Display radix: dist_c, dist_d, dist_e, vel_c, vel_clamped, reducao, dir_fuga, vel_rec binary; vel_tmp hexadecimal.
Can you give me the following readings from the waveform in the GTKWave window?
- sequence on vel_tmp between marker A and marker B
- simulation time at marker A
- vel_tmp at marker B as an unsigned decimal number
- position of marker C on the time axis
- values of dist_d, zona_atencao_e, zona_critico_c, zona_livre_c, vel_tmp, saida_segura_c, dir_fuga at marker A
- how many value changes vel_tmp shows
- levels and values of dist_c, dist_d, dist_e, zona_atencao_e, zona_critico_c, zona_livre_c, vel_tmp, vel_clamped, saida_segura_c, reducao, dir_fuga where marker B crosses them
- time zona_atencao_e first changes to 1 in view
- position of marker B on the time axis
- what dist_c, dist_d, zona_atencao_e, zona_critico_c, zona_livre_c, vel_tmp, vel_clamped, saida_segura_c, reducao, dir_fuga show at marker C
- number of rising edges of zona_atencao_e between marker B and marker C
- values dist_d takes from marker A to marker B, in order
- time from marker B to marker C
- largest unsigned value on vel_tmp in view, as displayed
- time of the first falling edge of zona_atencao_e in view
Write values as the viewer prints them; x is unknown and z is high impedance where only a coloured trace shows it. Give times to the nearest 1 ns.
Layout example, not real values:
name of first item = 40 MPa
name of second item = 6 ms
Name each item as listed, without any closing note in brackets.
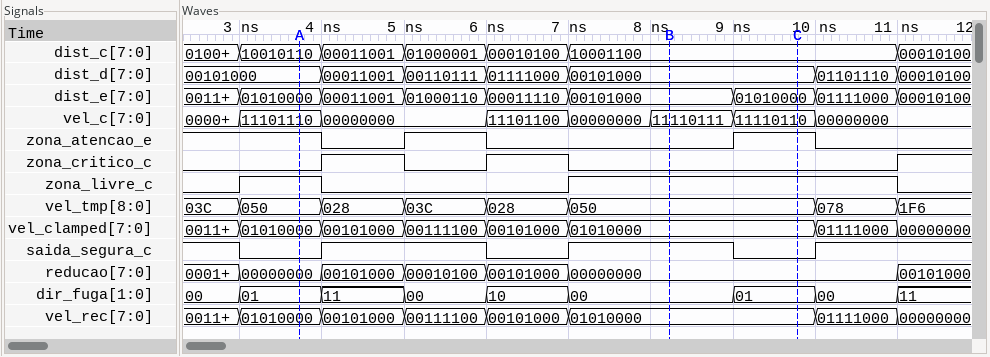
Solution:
sequence on vel_tmp between marker A and marker B = 050, 028, 03C, 028, 050
simulation time at marker A = 4 ns
vel_tmp at marker B as an unsigned decimal number = 80
position of marker C on the time axis = 10 ns
values of dist_d, zona_atencao_e, zona_critico_c, zona_livre_c, vel_tmp, saida_segura_c, dir_fuga at marker A = dist_d=00101000, zona_atencao_e=1, zona_critico_c=0, zona_livre_c=1, vel_tmp=050, saida_segura_c=0, dir_fuga=01
how many value changes vel_tmp shows = 7
levels and values of dist_c, dist_d, dist_e, zona_atencao_e, zona_critico_c, zona_livre_c, vel_tmp, vel_clamped, saida_segura_c, reducao, dir_fuga where marker B crosses them = dist_c=10001100, dist_d=00101000, dist_e=00101000, zona_atencao_e=0, zona_critico_c=0, zona_livre_c=1, vel_tmp=050, vel_clamped=01010000, saida_segura_c=1, reducao=00000000, dir_fuga=00
time zona_atencao_e first changes to 1 in view = 5 ns
position of marker B on the time axis = 8 ns
what dist_c, dist_d, zona_atencao_e, zona_critico_c, zona_livre_c, vel_tmp, vel_clamped, saida_segura_c, reducao, dir_fuga show at marker C = dist_c=10001100, dist_d=00101000, zona_atencao_e=1, zona_critico_c=0, zona_livre_c=1, vel_tmp=050, vel_clamped=01010000, saida_segura_c=0, reducao=00000000, dir_fuga=01
number of rising edges of zona_atencao_e between marker B and marker C = 1
values dist_d takes from marker A to marker B, in order = 00101000, 00011001, 00110111, 01111000, 00101000
time from marker B to marker C = 2 ns
largest unsigned value on vel_tmp in view, as displayed = 1F6
time of the first falling edge of zona_atencao_e in view = 4 ns
